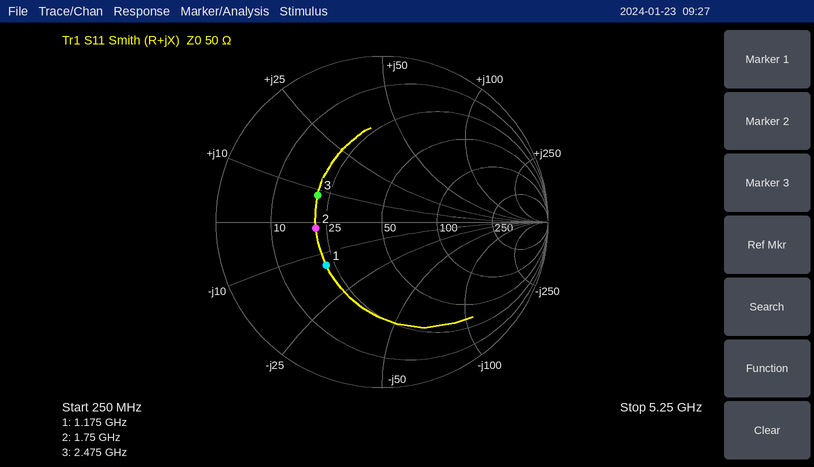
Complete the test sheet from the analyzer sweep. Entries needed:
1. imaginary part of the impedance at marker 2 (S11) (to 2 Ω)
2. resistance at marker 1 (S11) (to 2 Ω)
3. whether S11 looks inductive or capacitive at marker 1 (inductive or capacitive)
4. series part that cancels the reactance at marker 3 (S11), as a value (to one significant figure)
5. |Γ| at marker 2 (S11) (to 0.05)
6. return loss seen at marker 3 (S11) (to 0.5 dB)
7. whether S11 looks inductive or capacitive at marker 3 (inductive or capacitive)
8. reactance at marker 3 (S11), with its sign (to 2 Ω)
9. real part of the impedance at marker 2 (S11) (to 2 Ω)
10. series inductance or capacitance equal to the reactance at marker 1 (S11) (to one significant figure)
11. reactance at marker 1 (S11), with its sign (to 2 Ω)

-2 Ω
22 Ω
capacitive
8 pF
0.40
7.5 dB
inductive
+8 Ω
22 Ω
10 pF
-14 Ω
